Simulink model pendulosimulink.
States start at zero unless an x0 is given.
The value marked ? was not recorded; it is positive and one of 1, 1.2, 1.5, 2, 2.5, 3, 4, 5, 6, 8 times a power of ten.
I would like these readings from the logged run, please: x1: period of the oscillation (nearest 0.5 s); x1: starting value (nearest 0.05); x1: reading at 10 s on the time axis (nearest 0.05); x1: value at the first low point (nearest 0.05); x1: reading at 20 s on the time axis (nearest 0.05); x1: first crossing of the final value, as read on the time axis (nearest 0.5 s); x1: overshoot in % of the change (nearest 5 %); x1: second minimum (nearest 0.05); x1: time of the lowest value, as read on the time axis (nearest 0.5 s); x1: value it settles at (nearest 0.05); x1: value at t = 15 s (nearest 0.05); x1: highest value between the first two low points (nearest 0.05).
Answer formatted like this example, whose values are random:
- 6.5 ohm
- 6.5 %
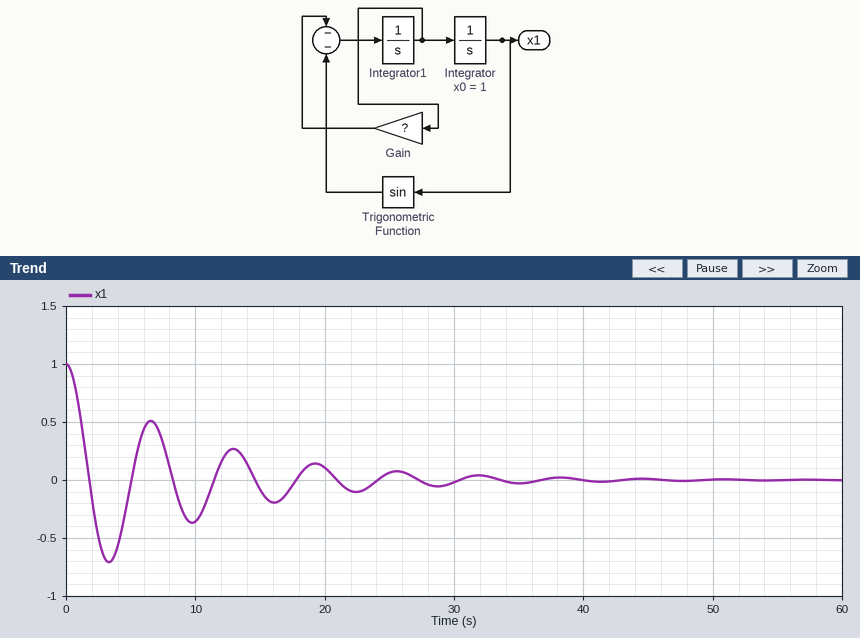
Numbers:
- 6.5 s
- 1.00
- -0.35
- -0.70
- 0.10
- 2.0 s
- 70 %
- -0.35
- 3.5 s
- 0.00
- -0.10
- 0.50
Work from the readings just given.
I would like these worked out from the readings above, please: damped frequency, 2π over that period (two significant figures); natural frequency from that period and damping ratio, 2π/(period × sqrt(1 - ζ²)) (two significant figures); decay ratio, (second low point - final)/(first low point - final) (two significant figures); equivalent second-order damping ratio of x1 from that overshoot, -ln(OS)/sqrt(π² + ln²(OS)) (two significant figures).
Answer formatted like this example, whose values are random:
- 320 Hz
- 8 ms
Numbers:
- 0.97 rad/s
- 0.97 rad/s
- 0.50
- 0.11
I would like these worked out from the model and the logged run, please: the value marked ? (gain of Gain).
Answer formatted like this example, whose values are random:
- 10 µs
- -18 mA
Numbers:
- 0.2
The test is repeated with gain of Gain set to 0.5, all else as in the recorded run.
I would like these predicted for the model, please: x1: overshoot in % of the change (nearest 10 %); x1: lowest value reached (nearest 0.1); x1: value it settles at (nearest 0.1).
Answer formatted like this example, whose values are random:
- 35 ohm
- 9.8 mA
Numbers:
- 40 %
- -0.4
- 0.0
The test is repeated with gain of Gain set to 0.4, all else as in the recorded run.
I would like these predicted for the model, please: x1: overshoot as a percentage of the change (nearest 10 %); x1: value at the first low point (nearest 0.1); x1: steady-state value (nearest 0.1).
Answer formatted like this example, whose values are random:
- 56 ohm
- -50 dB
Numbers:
- 50 %
- -0.5
- 0.0
